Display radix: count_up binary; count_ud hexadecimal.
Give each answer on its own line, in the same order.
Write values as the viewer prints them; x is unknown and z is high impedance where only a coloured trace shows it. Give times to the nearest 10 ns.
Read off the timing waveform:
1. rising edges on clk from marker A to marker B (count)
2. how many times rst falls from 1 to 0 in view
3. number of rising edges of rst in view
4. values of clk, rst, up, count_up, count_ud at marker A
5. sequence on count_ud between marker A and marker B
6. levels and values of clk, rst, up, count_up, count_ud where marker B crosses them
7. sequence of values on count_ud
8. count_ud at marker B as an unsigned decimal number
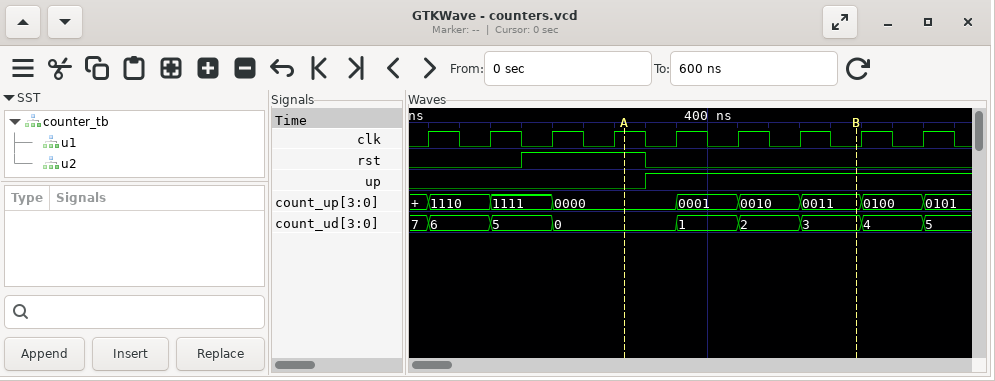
3
1
1
clk=1, rst=1, up=0, count_up=0000, count_ud=0
0, 1, 2, 3
clk=0, rst=0, up=1, count_up=0011, count_ud=3
7, 6, 5, 0, 1, 2, 3, 4, 5
3
